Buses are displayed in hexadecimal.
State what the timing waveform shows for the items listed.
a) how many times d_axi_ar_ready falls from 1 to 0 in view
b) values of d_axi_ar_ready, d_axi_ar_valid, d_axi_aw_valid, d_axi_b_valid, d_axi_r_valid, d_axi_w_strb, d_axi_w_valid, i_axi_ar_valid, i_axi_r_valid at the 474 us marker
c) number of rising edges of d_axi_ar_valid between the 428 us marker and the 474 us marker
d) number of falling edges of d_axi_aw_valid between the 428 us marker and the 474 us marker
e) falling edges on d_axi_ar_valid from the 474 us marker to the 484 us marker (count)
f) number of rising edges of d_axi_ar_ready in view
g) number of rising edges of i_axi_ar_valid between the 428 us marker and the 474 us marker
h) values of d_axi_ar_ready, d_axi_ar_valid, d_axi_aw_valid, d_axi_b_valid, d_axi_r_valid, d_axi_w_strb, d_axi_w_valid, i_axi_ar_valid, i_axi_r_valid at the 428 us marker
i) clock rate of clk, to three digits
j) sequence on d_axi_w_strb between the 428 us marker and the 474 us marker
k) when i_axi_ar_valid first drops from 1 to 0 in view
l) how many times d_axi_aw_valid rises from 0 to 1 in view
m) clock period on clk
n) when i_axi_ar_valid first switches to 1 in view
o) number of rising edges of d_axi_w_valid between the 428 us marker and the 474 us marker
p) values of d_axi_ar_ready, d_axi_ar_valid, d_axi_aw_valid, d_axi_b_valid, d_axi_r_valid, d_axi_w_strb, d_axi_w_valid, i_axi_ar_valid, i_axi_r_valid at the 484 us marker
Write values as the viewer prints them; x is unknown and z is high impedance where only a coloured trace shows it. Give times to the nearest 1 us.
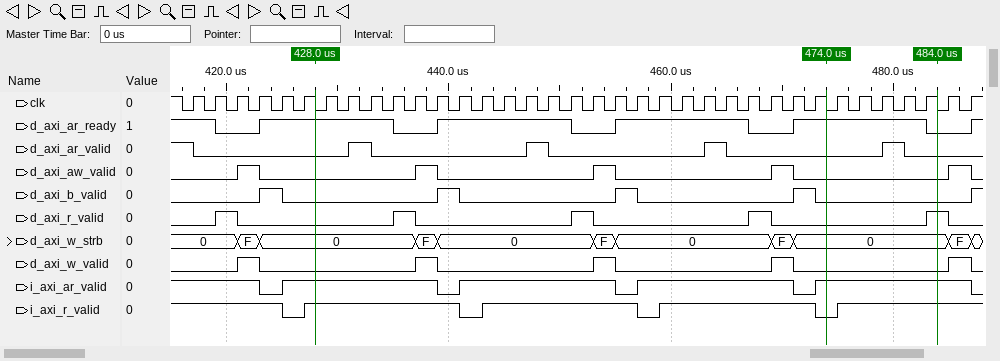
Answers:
5
d_axi_ar_ready=1, d_axi_ar_valid=0, d_axi_aw_valid=0, d_axi_b_valid=0, d_axi_r_valid=0, d_axi_w_strb=0, d_axi_w_valid=0, i_axi_ar_valid=1, i_axi_r_valid=0
3
3
1
5
3
d_axi_ar_ready=1, d_axi_ar_valid=0, d_axi_aw_valid=0, d_axi_b_valid=0, d_axi_r_valid=0, d_axi_w_strb=0, d_axi_w_valid=0, i_axi_ar_valid=1, i_axi_r_valid=1
500 kHz
0, F, 0, F, 0, F, 0
423 us
5
2 us
425 us
3
d_axi_ar_ready=0, d_axi_ar_valid=0, d_axi_aw_valid=0, d_axi_b_valid=0, d_axi_r_valid=1, d_axi_w_strb=0, d_axi_w_valid=0, i_axi_ar_valid=1, i_axi_r_valid=1
